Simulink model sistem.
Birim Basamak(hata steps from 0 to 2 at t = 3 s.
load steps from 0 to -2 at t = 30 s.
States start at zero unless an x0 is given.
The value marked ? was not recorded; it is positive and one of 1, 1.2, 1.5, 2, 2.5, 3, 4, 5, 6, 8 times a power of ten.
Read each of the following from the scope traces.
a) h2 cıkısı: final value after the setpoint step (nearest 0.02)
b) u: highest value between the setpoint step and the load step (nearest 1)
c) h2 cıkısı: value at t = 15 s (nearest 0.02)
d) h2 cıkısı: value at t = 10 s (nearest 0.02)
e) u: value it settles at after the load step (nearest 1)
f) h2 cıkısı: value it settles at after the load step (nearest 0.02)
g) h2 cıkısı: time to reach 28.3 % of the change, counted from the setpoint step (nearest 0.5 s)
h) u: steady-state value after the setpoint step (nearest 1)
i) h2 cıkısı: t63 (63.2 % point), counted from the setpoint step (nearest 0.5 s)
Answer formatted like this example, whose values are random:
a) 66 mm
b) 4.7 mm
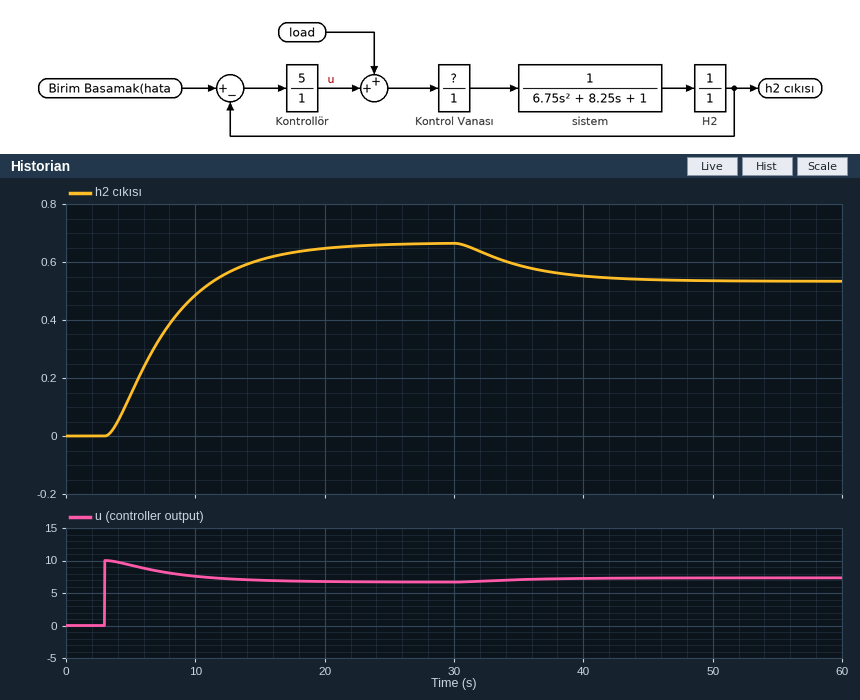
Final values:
a) 0.66
b) 10
c) 0.60
d) 0.48
e) 7
f) 0.54
g) 2.5 s
h) 7
i) 5.5 s
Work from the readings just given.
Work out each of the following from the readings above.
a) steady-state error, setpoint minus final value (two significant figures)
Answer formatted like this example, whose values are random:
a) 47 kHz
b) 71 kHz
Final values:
a) 1.3
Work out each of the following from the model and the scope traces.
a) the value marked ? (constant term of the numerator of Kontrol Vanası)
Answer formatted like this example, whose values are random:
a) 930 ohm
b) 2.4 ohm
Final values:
a) 0.1
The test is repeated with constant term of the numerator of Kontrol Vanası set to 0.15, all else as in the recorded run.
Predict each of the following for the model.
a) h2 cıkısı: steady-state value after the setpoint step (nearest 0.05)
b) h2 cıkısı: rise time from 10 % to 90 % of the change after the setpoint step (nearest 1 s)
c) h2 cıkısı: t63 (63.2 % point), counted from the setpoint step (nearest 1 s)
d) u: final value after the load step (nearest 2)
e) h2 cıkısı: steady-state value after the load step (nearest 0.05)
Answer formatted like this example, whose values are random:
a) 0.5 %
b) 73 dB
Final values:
a) 0.85
b) 9 s
c) 5 s
d) 6
e) 0.70
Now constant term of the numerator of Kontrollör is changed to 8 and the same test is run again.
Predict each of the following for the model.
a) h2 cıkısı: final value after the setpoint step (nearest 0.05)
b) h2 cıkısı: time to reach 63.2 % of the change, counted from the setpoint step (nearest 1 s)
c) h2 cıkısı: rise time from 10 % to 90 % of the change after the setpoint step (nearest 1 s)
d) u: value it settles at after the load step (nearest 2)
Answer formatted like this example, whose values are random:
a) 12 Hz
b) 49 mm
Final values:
a) 0.90
b) 5 s
c) 8 s
d) 10
